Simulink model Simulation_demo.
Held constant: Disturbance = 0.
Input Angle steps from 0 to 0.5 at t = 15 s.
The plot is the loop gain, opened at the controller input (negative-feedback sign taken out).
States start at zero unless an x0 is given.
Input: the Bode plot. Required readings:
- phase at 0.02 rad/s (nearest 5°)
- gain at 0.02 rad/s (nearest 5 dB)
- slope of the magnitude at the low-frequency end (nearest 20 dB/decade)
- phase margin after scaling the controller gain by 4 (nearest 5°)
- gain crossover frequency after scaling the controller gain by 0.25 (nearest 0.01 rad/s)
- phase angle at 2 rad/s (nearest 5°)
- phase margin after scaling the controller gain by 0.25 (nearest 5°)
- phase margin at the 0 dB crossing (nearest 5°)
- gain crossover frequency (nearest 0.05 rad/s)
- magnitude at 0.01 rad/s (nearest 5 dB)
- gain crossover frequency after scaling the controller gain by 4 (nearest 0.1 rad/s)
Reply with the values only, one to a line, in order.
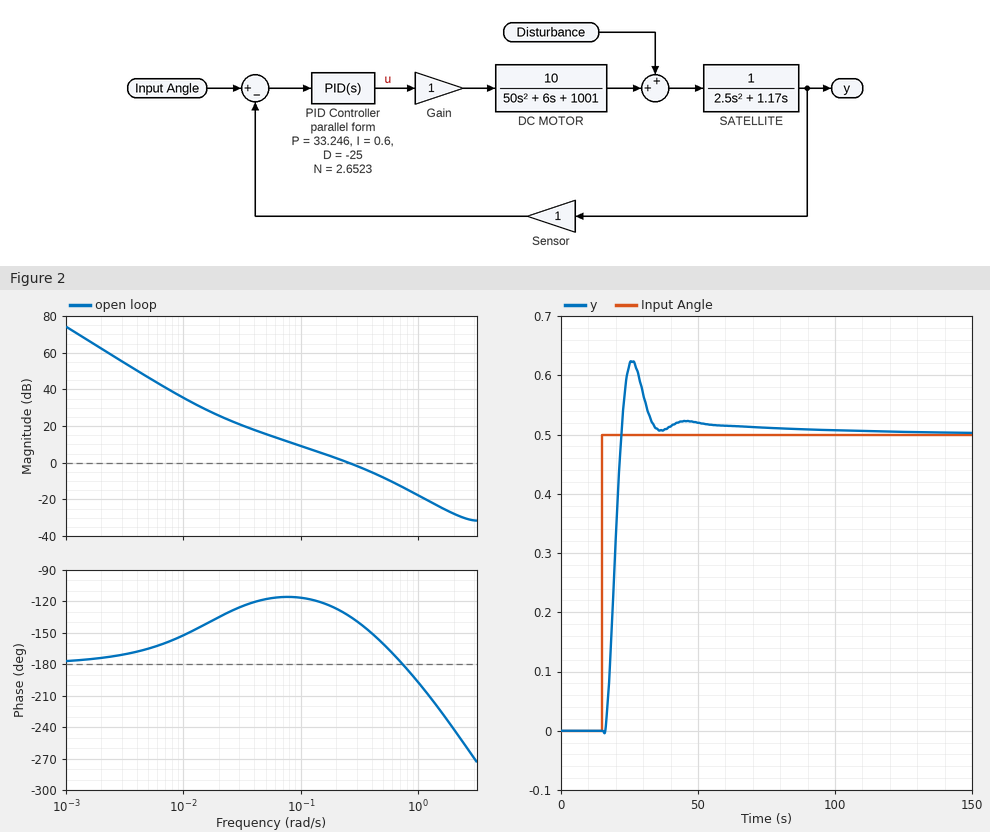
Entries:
-135°
25 dB
-40 dB/decade
5°
0.07 rad/s
-240°
65°
45°
0.25 rad/s
35 dB
0.7 rad/s
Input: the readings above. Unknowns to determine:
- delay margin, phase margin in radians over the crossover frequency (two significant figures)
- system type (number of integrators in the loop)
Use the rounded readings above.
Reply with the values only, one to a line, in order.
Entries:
3.1 s
2
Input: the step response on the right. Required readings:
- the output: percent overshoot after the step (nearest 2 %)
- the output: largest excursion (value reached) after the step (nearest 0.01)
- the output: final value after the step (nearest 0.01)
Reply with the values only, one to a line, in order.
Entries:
24 %
0.62
0.50
